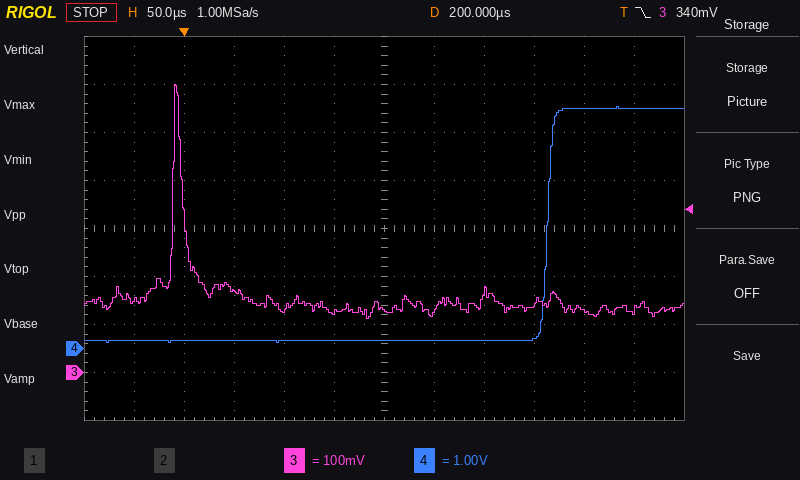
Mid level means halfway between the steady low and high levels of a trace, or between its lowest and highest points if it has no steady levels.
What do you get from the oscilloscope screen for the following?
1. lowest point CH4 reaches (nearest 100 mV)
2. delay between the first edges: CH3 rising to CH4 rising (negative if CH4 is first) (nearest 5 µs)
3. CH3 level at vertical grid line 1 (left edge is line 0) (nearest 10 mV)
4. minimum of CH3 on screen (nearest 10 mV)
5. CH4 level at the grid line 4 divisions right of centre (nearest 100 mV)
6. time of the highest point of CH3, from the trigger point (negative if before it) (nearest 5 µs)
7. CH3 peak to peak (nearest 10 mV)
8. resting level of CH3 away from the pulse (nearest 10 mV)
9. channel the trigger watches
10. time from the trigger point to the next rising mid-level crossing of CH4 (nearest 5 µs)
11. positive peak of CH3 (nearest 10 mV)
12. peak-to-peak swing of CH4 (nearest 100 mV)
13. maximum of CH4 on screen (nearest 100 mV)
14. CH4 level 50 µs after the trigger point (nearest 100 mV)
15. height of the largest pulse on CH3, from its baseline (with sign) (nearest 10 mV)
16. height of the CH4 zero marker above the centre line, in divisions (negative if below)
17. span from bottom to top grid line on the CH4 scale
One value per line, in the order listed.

100 mV
+375 µs
150 mV
110 mV
5.0 V
-10 µs
490 mV
140 mV
CH3
365 µs
600 mV
4.9 V
5.0 V
200 mV
+460 mV
-2.5 div
8 V
